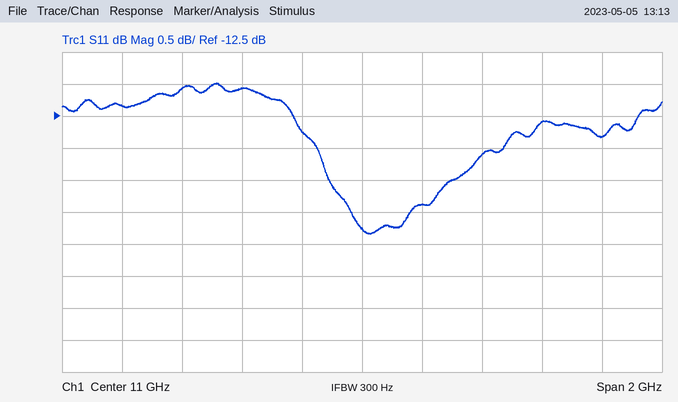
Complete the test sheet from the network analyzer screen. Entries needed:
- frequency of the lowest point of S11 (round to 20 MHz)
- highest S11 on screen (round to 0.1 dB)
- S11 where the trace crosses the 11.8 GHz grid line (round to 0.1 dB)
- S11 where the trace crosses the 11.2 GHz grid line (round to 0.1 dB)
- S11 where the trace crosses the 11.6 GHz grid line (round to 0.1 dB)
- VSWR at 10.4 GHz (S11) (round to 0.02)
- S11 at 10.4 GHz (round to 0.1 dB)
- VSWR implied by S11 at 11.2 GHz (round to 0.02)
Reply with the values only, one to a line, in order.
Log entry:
11.02 GHz
-12.0 dB
-12.8 dB
-13.9 dB
-12.6 dB
1.66
-12.1 dB
1.50
